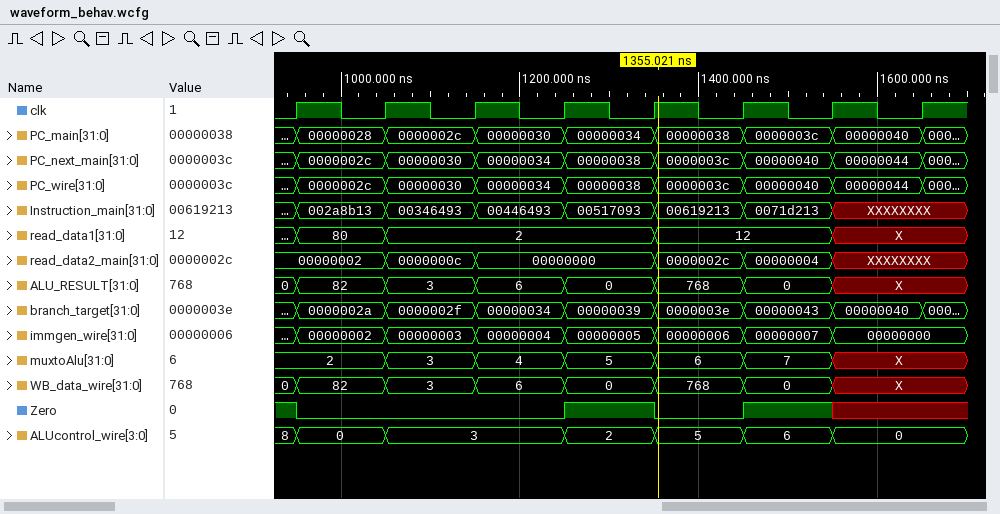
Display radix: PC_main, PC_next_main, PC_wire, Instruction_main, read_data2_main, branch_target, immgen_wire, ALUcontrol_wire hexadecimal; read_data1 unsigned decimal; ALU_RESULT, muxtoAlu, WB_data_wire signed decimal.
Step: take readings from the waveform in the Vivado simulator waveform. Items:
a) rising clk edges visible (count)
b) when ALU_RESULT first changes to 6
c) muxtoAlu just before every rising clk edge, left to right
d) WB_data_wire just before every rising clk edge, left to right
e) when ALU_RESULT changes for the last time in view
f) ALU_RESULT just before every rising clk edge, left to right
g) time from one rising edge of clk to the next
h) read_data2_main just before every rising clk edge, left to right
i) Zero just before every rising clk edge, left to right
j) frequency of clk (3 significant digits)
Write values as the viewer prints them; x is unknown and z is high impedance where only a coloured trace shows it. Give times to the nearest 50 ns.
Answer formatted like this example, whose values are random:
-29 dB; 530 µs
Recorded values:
8; 1150 ns; 2, 2, 3, 4, 5, 6, 7, X; 0, 82, 3, 6, 0, 768, 0, X; 1550 ns; 0, 82, 3, 6, 0, 768, 0, X; 100 ns; 00000002, 00000002, 0000000c, 00000000, 00000000, 0000002c, 00000004, XXXXXXXX; 1 0 0 0 1 0 1 x; 10.0 MHz
